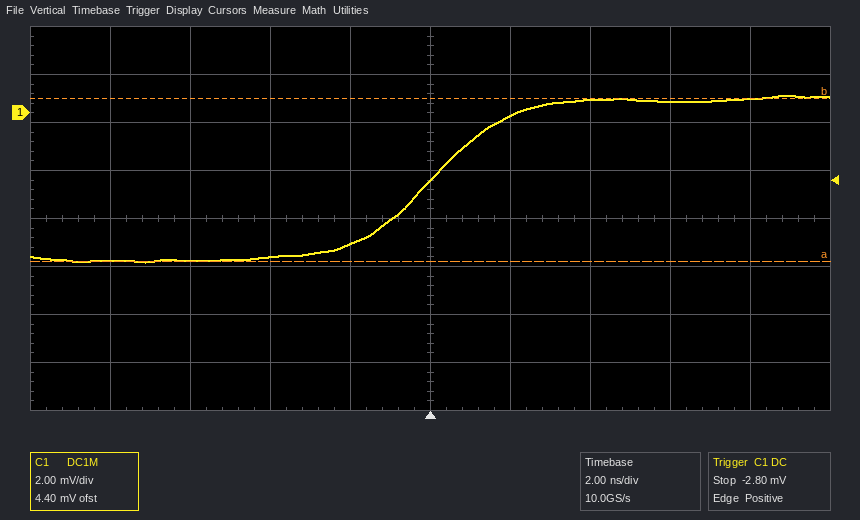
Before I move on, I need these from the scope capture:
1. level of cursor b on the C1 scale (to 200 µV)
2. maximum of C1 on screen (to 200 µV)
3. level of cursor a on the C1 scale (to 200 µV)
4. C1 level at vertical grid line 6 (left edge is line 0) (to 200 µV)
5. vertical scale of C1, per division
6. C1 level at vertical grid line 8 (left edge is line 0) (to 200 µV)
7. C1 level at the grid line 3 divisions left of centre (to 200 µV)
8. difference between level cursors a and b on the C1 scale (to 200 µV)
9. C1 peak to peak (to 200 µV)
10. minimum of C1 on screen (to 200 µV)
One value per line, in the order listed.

600 µV
800 µV
-6.2 mV
-200 µV
2 mV
400 µV
-6.2 mV
6.8 mV
7.0 mV
-6.2 mV
